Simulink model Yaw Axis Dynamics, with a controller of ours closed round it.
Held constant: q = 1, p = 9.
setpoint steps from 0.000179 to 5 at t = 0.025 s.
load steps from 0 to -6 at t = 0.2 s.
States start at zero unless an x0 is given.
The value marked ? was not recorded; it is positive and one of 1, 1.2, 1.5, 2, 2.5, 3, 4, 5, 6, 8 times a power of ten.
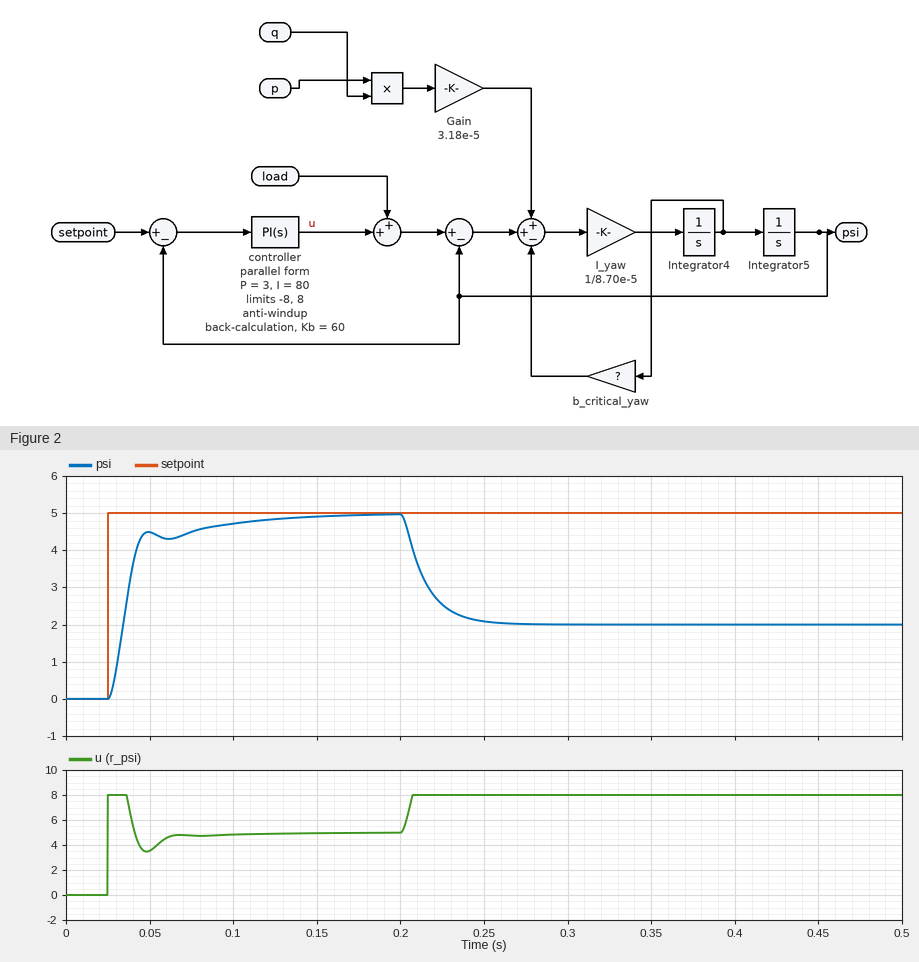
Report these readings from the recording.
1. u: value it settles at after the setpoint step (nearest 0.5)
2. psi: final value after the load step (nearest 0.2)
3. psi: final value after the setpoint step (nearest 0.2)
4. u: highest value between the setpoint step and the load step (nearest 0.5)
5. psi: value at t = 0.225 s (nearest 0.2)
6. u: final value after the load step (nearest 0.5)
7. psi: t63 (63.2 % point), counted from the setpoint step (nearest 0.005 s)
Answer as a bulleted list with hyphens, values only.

- 5.0
- 2.0
- 5.0
- 8.0
- 2.6
- 8.0
- 0.015 s
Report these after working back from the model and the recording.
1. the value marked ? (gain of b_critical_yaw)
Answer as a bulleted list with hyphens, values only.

- 0.02
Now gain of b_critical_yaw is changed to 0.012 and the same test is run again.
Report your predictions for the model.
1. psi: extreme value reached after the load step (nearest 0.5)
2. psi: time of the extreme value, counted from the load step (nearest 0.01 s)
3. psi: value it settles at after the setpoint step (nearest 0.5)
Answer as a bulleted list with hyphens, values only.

- 1.5
- 0.03 s
- 5.0
